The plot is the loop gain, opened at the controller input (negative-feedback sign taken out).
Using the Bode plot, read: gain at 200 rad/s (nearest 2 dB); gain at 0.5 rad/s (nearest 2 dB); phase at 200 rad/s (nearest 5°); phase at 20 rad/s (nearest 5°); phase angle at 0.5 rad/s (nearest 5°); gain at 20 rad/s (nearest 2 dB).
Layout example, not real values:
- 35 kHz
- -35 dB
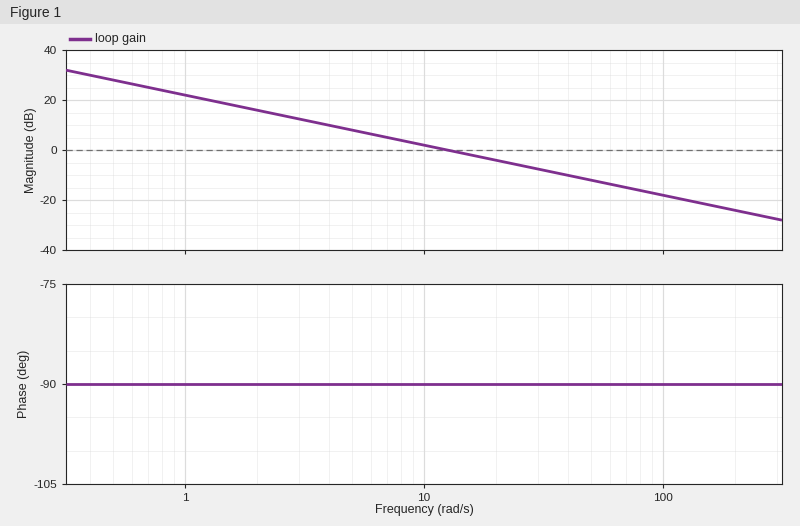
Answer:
- -24 dB
- 28 dB
- -90°
- -90°
- -90°
- -4 dB
